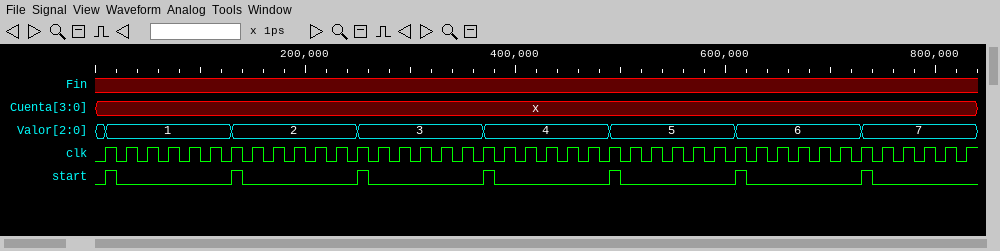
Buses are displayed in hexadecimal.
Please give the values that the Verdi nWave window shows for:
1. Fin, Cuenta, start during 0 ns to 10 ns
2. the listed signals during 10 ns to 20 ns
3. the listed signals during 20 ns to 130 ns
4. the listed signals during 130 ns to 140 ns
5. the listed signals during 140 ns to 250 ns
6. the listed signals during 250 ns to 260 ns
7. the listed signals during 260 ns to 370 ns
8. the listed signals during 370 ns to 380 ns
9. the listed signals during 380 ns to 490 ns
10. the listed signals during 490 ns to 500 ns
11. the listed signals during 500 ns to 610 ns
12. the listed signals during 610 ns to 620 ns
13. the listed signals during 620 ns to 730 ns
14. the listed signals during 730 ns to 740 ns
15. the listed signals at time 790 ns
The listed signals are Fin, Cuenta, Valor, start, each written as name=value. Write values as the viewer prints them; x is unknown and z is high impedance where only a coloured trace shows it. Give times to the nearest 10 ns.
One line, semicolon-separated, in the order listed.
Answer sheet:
Fin=x, Cuenta=x, start=0; Fin=x, Cuenta=x, Valor=1, start=1; Fin=x, Cuenta=x, Valor=1, start=0; Fin=x, Cuenta=x, Valor=2, start=1; Fin=x, Cuenta=x, Valor=2, start=0; Fin=x, Cuenta=x, Valor=3, start=1; Fin=x, Cuenta=x, Valor=3, start=0; Fin=x, Cuenta=x, Valor=4, start=1; Fin=x, Cuenta=x, Valor=4, start=0; Fin=x, Cuenta=x, Valor=5, start=1; Fin=x, Cuenta=x, Valor=5, start=0; Fin=x, Cuenta=x, Valor=6, start=1; Fin=x, Cuenta=x, Valor=6, start=0; Fin=x, Cuenta=x, Valor=7, start=1; Fin=x, Cuenta=x, Valor=7, start=0
